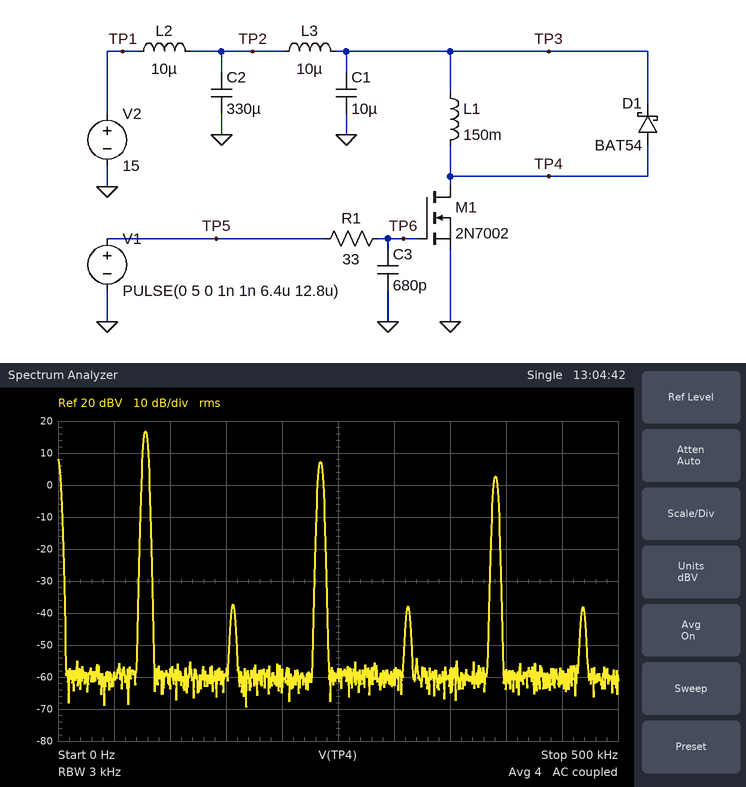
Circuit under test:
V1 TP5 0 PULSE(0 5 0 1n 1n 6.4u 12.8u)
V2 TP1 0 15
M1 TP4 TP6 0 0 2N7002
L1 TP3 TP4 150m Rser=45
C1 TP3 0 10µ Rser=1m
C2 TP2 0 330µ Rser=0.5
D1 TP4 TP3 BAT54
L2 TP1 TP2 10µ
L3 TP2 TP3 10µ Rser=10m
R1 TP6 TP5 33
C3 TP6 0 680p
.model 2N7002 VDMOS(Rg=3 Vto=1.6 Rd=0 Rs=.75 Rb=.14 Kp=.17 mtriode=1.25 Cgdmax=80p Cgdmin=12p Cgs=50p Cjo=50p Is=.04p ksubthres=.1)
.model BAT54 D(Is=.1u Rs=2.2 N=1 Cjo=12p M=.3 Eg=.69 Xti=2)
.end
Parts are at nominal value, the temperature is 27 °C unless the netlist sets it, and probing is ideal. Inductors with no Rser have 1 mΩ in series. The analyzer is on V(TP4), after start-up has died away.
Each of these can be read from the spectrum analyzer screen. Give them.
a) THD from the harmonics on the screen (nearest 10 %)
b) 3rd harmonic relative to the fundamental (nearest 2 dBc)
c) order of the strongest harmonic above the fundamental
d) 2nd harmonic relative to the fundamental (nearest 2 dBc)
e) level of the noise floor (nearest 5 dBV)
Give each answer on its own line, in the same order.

40 %
-10 dBc
3
-54 dBc
-60 dBV
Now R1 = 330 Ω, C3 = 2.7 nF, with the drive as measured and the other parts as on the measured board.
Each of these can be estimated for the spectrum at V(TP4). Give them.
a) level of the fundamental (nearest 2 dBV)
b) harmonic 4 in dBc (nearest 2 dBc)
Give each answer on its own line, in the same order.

16 dBV
-22 dBc
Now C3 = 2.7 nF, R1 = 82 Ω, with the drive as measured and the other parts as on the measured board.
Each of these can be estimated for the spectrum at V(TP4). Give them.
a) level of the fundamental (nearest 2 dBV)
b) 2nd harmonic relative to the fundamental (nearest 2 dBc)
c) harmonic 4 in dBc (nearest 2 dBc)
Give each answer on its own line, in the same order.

16 dBV
-32 dBc
-32 dBc
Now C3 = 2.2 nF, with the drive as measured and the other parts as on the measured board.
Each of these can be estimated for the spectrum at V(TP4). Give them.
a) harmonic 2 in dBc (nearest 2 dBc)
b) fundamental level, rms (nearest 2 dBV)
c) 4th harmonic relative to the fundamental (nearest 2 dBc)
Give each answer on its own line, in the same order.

-42 dBc
16 dBV
-42 dBc
